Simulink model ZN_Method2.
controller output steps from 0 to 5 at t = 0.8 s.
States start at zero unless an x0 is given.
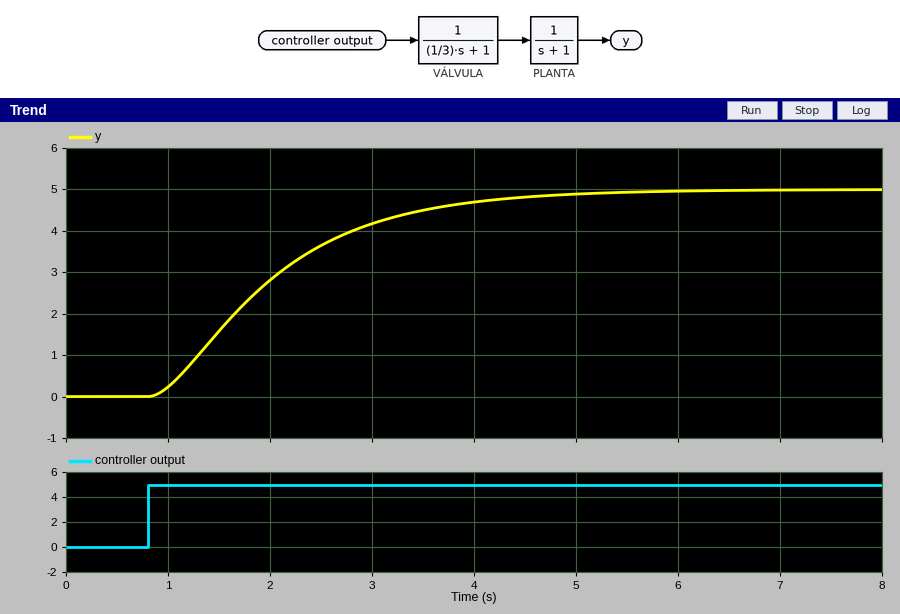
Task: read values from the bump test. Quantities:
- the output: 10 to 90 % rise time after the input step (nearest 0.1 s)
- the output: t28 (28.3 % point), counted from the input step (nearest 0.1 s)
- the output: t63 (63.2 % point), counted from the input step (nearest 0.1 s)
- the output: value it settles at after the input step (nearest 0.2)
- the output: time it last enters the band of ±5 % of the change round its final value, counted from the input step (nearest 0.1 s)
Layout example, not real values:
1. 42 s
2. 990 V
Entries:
1. 2.4 s
2. 0.6 s
3. 1.4 s
4. 5.0
5. 3.4 s
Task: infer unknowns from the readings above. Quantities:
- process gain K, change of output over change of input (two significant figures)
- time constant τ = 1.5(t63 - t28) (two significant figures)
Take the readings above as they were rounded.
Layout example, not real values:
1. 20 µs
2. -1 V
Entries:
1. 1.0
2. 1.2 s
